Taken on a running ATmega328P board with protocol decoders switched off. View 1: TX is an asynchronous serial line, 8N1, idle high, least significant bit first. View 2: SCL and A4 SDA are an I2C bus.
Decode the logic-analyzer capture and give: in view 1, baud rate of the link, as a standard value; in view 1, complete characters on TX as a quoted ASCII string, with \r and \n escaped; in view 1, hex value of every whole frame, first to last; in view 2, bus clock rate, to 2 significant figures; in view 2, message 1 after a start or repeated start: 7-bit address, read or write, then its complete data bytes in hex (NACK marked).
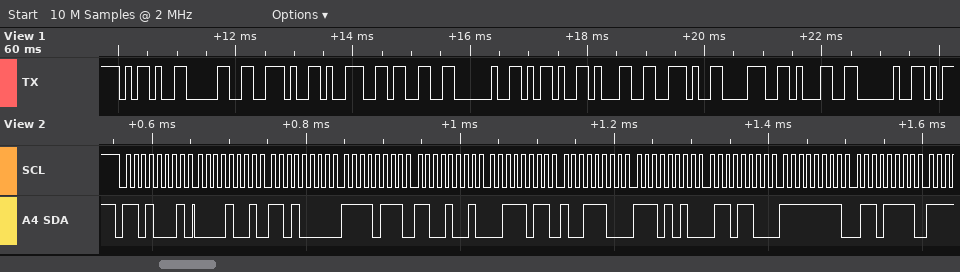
9600 baud
"-0.93 -1.81 "
0x2D 0x30 0x2E 0x39 0x33 0x20 0x2D 0x31 0x2E 0x38 0x31 0x20
100 kHz
0x68 read: 09 D0 F7 C9 3B 9C EA 6C FF 6F
